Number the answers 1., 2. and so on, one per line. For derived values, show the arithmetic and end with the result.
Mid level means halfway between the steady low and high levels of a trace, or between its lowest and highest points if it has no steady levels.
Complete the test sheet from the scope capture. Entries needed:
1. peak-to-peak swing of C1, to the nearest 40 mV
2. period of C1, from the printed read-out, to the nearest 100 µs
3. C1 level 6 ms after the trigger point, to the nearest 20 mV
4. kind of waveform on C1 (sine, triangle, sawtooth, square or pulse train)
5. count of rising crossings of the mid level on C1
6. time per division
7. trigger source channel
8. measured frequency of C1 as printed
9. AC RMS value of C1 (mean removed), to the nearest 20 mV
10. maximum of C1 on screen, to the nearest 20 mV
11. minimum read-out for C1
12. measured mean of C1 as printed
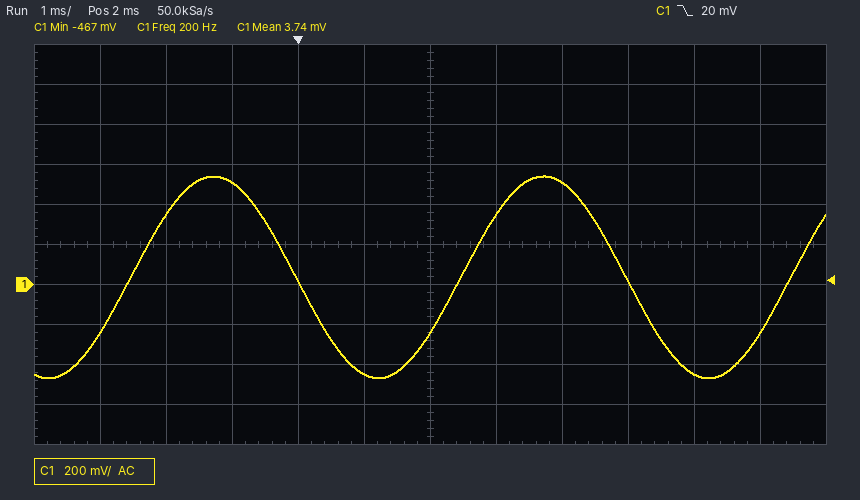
1. 1.00 V
2. 1 / 200 Hz ≈ 5.0 ms
3. -440 mV
4. sine
5. 3
6. 1 ms
7. C1
8. 200 Hz
9. 1.00 V / (2√2) ≈ 354 mV, so 360 mV to the nearest 20 mV
10. 540 mV
11. -467 mV
12. 3.74 mV
